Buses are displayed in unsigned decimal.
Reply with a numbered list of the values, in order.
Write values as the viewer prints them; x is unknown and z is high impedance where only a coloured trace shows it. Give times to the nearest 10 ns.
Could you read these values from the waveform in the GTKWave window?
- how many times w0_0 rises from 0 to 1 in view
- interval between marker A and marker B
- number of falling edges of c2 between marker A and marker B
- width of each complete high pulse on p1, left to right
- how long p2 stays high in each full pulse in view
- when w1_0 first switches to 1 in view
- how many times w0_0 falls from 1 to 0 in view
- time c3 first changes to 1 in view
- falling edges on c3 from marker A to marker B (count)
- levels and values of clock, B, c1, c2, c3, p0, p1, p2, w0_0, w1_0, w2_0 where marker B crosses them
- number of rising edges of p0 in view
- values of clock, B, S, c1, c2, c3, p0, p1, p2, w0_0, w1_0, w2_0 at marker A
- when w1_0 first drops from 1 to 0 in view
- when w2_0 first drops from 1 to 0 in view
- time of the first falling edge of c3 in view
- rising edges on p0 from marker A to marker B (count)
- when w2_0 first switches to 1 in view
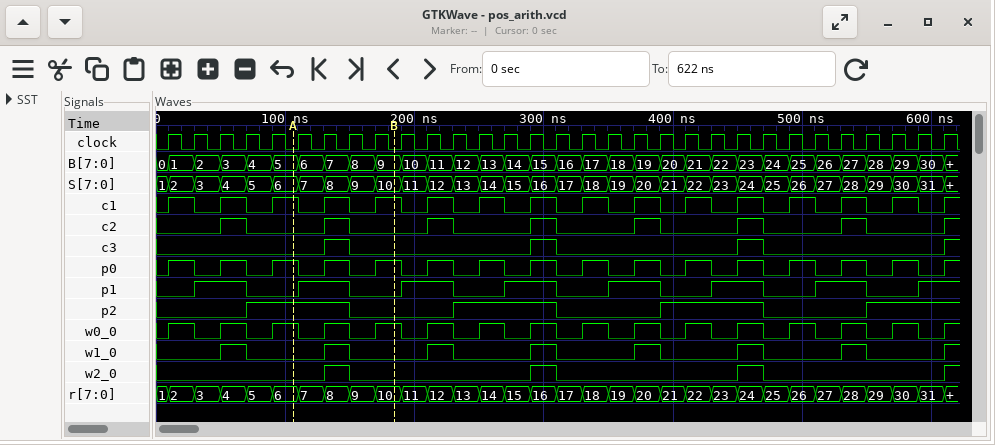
1. 16
2. 80 ns
3. 1
4. 40 ns, 40 ns, 40 ns, 40 ns, 40 ns, 40 ns, 40 ns
5. 80 ns, 80 ns, 80 ns
6. 50 ns
7. 15
8. 130 ns
9. 1
10. clock=0, B=9, c1=1, c2=0, c3=0, p0=1, p1=0, p2=0, w0_0=1, w1_0=0, w2_0=0
11. 16
12. clock=0, B=5, S=6, c1=1, c2=0, c3=0, p0=1, p1=0, p2=1, w0_0=1, w1_0=0, w2_0=0
13. 70 ns
14. 150 ns
15. 150 ns
16. 2
17. 130 ns
